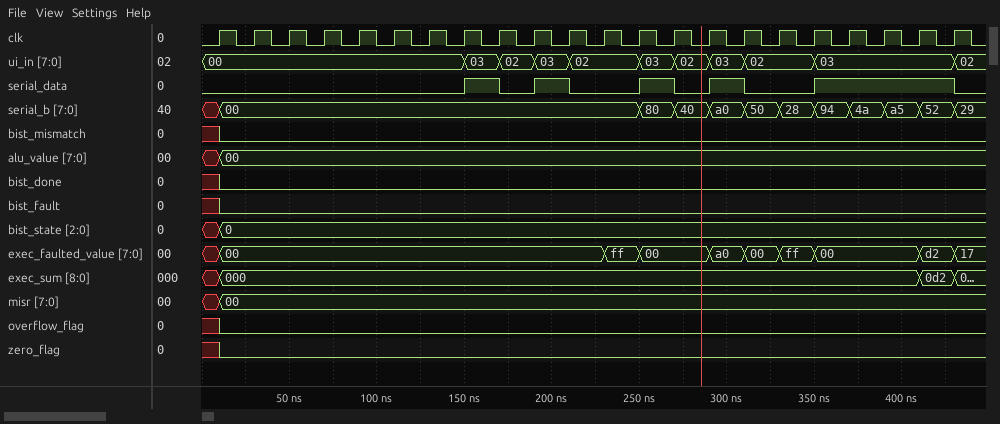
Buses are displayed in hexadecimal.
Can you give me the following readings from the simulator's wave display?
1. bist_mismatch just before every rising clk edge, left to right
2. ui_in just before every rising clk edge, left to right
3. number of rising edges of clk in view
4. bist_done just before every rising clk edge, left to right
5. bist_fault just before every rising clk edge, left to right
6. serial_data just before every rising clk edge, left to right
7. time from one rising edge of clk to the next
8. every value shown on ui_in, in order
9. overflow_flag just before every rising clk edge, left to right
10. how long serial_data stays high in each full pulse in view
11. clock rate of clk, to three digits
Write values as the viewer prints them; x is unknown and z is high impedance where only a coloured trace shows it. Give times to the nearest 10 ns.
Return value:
x 0 0 0 0 0 0 0 0 0 0 0 0 0 0 0 0 0 0 0 0 0
00, 00, 00, 00, 00, 00, 00, 00, 03, 02, 03, 02, 02, 03, 02, 03, 02, 02, 03, 03, 03, 03
22
x 0 0 0 0 0 0 0 0 0 0 0 0 0 0 0 0 0 0 0 0 0
x 0 0 0 0 0 0 0 0 0 0 0 0 0 0 0 0 0 0 0 0 0
0 0 0 0 0 0 0 0 1 0 1 0 0 1 0 1 0 0 1 1 1 1
20 ns
00, 03, 02, 03, 02, 03, 02, 03, 02, 03, 02
x 0 0 0 0 0 0 0 0 0 0 0 0 0 0 0 0 0 0 0 0 0
20 ns, 20 ns, 20 ns, 20 ns, 80 ns
50.0 MHz
